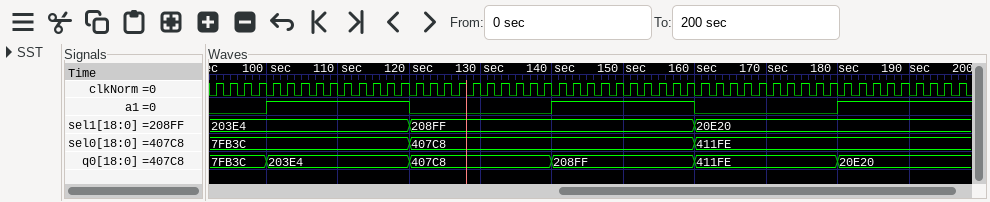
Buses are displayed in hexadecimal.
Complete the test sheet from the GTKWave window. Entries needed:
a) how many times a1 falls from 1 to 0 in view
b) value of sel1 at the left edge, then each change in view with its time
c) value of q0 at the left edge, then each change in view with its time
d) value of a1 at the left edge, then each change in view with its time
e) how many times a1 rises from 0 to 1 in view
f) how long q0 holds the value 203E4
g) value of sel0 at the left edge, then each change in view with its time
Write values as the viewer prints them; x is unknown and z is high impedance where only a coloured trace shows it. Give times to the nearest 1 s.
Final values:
2
203E4, 208FF at 120 s, 20E20 at 160 s
7FB3C, 203E4 at 100 s, 407C8 at 120 s, 208FF at 140 s, 411FE at 160 s, 20E20 at 180 s
0, 1 at 100 s, 0 at 120 s, 1 at 140 s, 0 at 160 s, 1 at 180 s
3
20 s
7FB3C, 407C8 at 120 s, 411FE at 160 s
